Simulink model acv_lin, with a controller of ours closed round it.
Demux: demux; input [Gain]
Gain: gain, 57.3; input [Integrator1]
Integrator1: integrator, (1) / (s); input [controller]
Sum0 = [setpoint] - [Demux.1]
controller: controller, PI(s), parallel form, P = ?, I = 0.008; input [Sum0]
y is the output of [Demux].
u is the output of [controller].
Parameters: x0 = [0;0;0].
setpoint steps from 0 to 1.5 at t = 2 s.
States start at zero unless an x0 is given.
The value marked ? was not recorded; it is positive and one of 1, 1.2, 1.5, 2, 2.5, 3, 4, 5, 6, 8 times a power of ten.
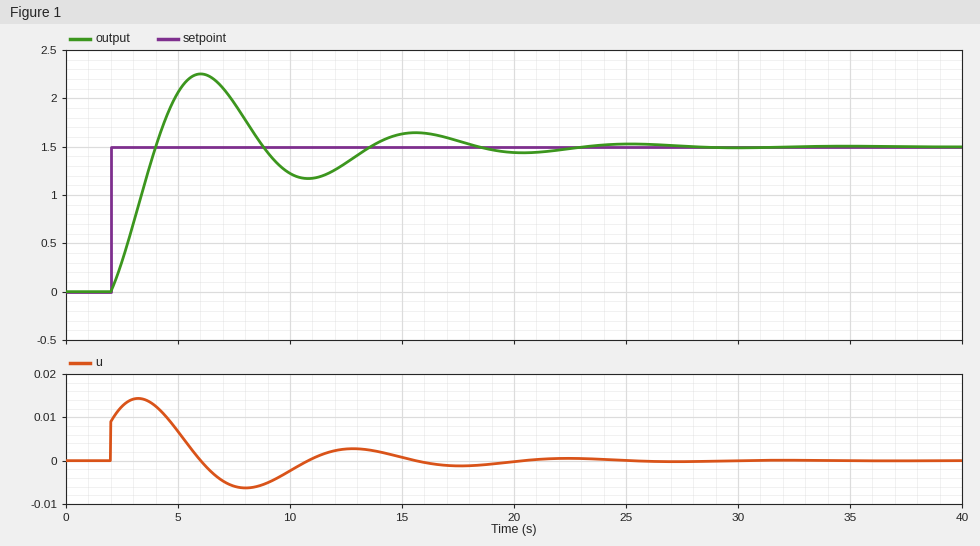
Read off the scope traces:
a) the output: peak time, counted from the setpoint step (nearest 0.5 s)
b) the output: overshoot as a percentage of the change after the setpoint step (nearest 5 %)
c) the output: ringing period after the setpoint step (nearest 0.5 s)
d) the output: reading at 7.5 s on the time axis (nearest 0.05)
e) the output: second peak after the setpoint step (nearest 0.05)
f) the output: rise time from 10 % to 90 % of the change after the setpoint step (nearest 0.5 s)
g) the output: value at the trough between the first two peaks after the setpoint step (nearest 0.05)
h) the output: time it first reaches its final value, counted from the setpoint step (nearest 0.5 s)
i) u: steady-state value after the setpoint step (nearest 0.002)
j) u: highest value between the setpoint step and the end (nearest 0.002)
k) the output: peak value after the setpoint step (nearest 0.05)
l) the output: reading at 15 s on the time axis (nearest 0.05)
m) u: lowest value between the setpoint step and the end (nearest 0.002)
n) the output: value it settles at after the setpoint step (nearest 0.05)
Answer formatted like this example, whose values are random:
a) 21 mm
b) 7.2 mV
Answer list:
a) 4.0 s
b) 50 %
c) 9.5 s
d) 1.95
e) 1.65
f) 1.5 s
g) 1.15
h) 2.0 s
i) 0.000
j) 0.014
k) 2.25
l) 1.65
m) -0.006
n) 1.50
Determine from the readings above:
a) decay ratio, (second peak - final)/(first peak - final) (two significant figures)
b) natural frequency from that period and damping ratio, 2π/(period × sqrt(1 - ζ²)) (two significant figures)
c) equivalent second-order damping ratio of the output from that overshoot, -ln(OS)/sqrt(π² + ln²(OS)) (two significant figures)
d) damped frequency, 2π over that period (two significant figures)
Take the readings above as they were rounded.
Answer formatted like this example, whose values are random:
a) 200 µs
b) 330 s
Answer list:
a) 0.20
b) 0.68 rad/s
c) 0.22
d) 0.66 rad/s
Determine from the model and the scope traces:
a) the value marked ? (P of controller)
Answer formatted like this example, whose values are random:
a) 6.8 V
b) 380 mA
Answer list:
a) 0.006
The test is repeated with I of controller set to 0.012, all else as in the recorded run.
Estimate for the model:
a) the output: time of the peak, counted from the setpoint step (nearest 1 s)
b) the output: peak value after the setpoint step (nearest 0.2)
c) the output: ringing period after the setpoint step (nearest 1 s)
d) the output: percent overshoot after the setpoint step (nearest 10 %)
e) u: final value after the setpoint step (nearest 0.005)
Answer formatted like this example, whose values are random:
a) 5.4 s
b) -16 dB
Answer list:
a) 3 s
b) 2.4
c) 8 s
d) 60 %
e) 0.000
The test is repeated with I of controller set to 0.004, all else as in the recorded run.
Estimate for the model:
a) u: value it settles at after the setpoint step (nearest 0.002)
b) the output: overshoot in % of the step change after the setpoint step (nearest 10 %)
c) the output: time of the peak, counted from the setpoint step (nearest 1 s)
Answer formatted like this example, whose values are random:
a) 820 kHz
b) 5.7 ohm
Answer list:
a) 0.000
b) 40 %
c) 5 s
